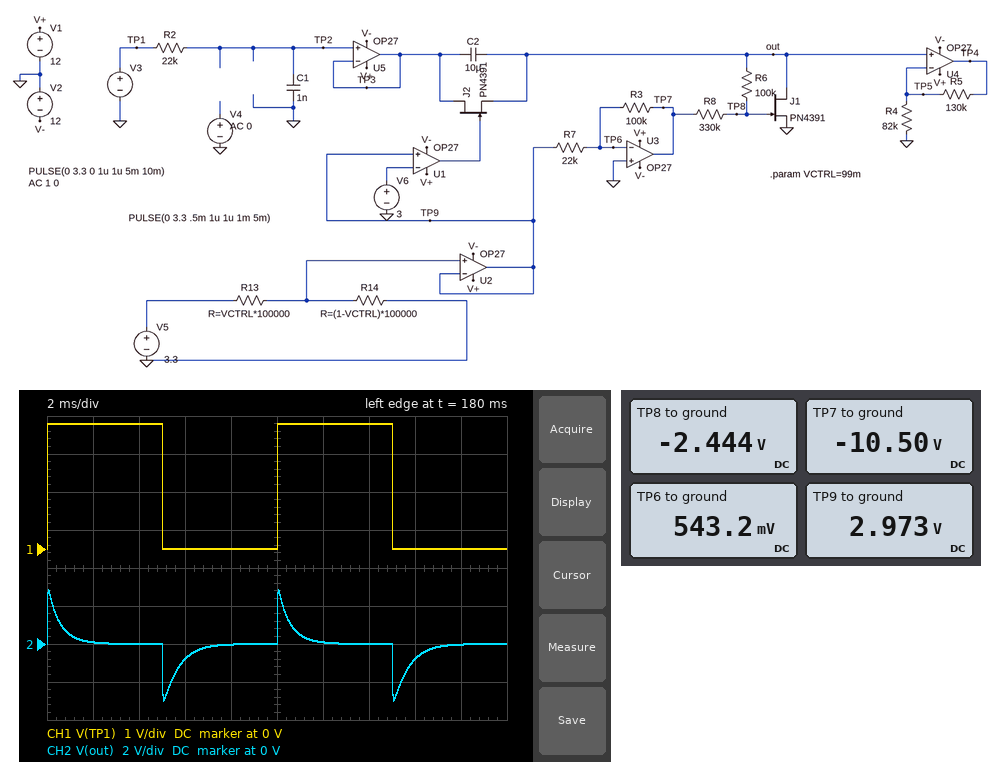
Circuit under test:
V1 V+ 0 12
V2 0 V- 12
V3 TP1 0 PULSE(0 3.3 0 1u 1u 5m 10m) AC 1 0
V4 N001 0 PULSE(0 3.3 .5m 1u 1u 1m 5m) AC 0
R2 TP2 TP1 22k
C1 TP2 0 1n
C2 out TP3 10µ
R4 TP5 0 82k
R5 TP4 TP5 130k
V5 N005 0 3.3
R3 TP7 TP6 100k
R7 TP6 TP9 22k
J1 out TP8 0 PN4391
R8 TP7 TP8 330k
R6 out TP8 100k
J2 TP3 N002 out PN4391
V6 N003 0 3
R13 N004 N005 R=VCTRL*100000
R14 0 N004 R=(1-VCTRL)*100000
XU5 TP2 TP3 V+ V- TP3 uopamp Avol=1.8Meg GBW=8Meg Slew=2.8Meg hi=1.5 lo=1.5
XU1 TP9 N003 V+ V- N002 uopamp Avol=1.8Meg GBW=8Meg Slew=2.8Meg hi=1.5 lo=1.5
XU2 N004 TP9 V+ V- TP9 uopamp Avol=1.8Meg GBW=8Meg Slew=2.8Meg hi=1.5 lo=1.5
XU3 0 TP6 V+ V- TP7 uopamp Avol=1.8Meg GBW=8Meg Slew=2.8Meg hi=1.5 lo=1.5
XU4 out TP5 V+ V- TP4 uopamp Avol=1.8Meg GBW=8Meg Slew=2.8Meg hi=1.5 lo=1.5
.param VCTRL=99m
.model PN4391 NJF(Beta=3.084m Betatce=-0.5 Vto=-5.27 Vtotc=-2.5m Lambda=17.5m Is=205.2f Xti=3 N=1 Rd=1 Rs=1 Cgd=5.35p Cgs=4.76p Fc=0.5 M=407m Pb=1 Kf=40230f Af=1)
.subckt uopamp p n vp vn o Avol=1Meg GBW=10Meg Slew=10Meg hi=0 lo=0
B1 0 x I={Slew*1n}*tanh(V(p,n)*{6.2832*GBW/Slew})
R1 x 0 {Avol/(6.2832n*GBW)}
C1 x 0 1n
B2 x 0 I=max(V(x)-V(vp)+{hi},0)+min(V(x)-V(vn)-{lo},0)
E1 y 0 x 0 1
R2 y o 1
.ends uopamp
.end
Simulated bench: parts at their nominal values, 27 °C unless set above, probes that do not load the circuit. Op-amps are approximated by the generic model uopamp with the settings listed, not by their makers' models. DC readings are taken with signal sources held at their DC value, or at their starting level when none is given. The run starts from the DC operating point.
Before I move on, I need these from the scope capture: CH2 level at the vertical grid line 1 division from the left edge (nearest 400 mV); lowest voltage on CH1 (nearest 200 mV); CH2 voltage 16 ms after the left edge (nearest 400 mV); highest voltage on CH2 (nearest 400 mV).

0 V
0 V
-800 mV
2.8 V
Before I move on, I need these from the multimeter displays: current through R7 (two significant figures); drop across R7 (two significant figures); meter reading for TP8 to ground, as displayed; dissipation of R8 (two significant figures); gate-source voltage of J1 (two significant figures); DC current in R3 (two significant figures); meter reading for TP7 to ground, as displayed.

110 µA
2.4 V
-2.444 V
200 µW
-2.4 V
110 µA
-10.50 V
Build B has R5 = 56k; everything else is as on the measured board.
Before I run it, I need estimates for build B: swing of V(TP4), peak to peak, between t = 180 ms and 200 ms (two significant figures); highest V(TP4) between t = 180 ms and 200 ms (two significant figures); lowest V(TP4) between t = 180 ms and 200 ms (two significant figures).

9.8 V
4.8 V
-5.0 V
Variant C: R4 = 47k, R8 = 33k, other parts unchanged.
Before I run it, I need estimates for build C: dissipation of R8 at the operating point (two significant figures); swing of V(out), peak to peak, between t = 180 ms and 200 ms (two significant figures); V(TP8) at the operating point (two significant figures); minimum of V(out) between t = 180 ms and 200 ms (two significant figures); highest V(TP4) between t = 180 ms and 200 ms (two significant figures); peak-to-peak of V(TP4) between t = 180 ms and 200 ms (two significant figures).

87 µW
3.3 V
-8.8 V
-3.8 V
-1.7 V
8.8 V
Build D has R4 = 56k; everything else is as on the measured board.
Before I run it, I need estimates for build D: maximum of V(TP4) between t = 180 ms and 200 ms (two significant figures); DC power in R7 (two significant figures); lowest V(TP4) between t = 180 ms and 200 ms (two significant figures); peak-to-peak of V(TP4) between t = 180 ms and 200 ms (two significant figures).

9.5 V
270 µW
-9.9 V
19 V
